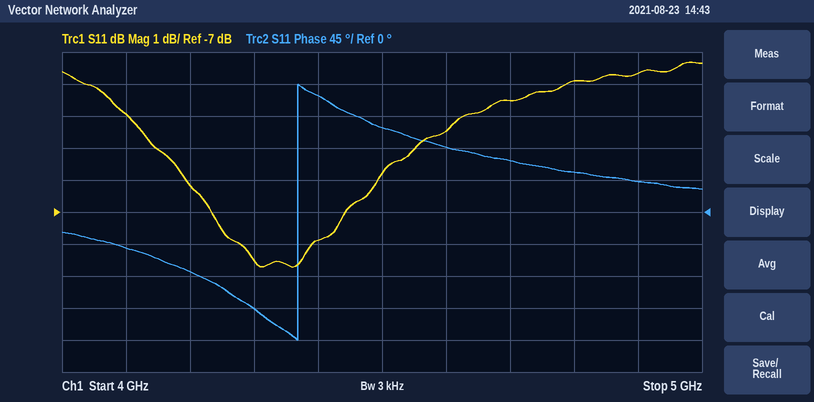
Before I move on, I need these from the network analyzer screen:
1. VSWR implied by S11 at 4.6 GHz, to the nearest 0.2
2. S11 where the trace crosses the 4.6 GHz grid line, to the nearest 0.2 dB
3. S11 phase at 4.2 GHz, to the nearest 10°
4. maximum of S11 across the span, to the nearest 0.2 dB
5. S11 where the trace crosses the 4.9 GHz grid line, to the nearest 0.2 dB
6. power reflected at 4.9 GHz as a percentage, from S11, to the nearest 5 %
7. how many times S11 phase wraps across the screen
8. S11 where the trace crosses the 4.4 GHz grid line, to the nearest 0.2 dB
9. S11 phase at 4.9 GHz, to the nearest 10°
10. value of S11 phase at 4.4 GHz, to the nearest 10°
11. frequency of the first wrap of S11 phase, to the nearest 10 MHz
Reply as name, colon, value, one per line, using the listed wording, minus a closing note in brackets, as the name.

VSWR implied by S11 at 4.6 GHz, to the nearest 0.2: 4.0
S11 where the trace crosses the 4.6 GHz grid line, to the nearest 0.2 dB: -4.4 dB
S11 phase at 4.2 GHz, to the nearest 10°: -80°
maximum of S11 across the span, to the nearest 0.2 dB: -2.4 dB
S11 where the trace crosses the 4.9 GHz grid line, to the nearest 0.2 dB: -2.6 dB
power reflected at 4.9 GHz as a percentage, from S11, to the nearest 5 %: 55 %
how many times S11 phase wraps across the screen: 1
S11 where the trace crosses the 4.4 GHz grid line, to the nearest 0.2 dB: -7.8 dB
S11 phase at 4.9 GHz, to the nearest 10°: 40°
value of S11 phase at 4.4 GHz, to the nearest 10°: 160°
frequency of the first wrap of S11 phase, to the nearest 10 MHz: 4.37 GHz
